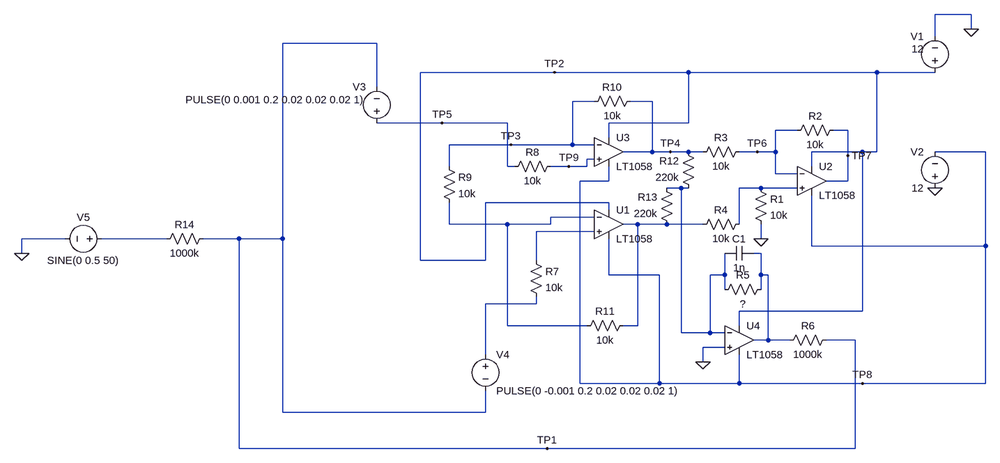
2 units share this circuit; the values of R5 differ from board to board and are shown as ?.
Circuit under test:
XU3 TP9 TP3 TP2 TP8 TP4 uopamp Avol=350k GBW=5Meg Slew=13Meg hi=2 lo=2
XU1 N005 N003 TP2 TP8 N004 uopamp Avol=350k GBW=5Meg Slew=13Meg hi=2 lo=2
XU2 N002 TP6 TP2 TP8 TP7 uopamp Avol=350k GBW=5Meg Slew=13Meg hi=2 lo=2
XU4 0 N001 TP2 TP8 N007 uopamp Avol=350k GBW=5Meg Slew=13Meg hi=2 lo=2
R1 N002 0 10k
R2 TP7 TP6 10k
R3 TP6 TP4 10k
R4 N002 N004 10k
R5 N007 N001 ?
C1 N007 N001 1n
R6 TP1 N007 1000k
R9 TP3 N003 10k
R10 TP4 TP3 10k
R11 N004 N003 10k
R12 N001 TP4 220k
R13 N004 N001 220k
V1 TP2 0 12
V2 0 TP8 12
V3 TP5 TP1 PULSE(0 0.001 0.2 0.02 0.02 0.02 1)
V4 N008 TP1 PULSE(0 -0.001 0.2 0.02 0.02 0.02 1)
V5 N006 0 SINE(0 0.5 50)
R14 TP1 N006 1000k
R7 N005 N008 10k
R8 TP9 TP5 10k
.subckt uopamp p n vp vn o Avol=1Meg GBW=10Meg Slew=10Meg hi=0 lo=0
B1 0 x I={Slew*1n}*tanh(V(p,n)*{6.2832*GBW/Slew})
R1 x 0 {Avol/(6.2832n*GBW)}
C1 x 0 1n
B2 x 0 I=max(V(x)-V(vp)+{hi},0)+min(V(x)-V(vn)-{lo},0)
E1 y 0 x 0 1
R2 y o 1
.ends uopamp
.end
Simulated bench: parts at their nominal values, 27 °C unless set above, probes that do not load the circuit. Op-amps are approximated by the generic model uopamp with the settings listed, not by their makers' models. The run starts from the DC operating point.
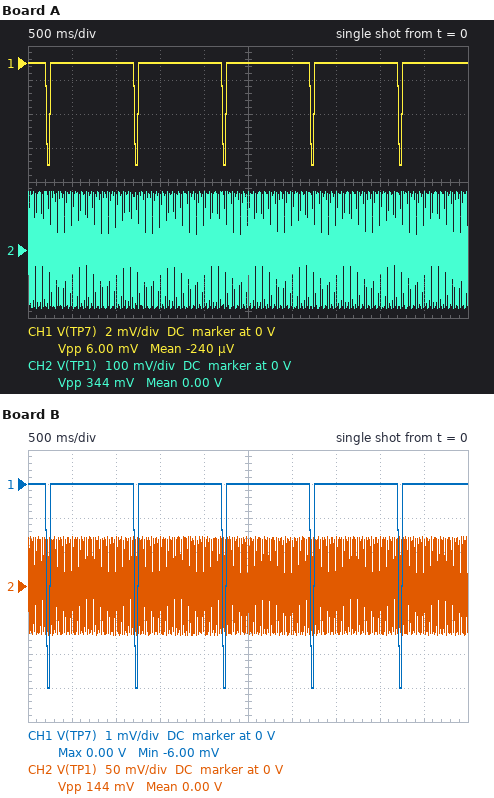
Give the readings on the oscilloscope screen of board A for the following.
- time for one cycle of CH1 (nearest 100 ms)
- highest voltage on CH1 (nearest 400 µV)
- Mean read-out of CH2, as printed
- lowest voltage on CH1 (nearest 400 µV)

1.0 s
0 V
0.00 V
-6.0 mV
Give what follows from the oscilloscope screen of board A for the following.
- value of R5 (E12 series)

100 kΩ
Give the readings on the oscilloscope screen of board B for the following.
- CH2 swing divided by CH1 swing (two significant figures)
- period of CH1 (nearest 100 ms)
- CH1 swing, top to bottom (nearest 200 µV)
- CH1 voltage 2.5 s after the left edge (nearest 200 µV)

24
1.0 s
6.0 mV
0 V
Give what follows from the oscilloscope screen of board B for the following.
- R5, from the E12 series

560 kΩ
